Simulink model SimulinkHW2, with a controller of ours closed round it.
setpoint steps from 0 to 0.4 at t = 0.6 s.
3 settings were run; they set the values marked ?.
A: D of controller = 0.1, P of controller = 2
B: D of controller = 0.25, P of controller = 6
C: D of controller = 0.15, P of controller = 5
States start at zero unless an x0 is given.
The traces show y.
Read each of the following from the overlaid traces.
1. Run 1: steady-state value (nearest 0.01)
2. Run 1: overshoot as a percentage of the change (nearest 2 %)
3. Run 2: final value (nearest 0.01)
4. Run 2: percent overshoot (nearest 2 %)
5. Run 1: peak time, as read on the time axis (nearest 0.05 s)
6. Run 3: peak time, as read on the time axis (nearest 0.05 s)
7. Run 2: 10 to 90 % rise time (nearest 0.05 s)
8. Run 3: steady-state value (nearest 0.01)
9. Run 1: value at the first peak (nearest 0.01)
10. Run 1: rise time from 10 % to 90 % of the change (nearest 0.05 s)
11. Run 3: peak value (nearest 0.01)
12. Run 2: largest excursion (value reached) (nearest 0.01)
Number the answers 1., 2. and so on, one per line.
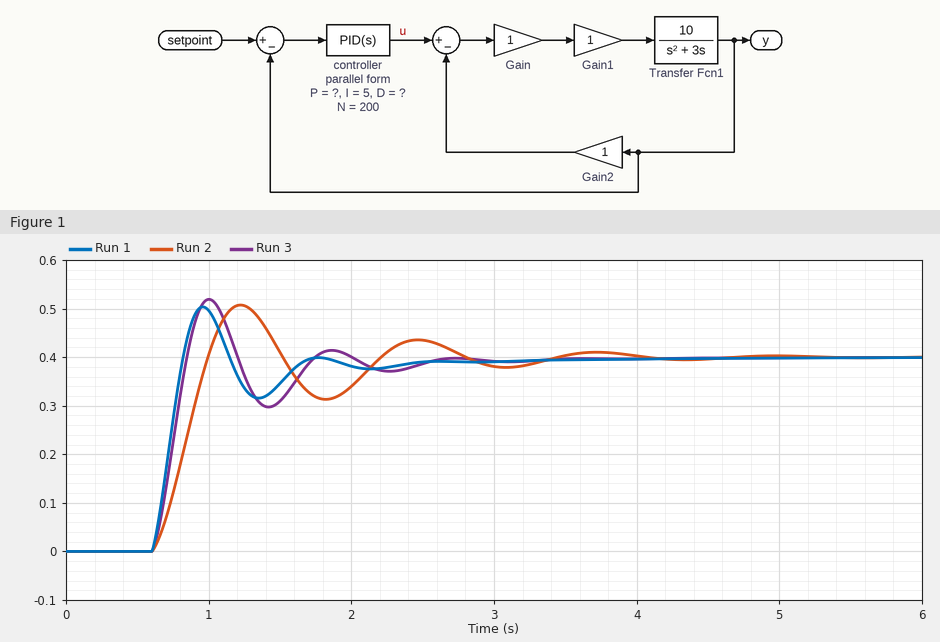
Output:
1. 0.40
2. 26 %
3. 0.40
4. 26 %
5. 0.95 s
6. 1.00 s
7. 0.30 s
8. 0.40
9. 0.50
10. 0.15 s
11. 0.52
12. 0.51
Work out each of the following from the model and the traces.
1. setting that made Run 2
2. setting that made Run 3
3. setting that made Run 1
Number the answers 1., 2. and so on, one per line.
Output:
1. A
2. C
3. B
